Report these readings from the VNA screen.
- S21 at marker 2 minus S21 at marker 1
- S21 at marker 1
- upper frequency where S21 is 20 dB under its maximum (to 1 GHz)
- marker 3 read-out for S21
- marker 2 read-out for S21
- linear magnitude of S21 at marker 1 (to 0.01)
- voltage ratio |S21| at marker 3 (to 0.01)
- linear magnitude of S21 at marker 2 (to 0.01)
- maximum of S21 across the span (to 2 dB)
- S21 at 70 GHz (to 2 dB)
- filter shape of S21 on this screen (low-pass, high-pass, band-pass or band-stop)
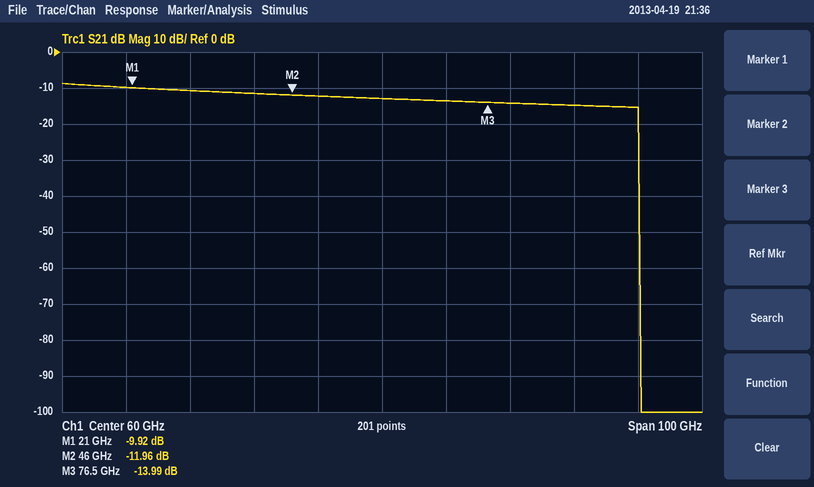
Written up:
-2.04 dB
-9.92 dB
100 GHz
-13.99 dB
-11.96 dB
0.32
0.20
0.25
-8 dB
-14 dB
low-pass
